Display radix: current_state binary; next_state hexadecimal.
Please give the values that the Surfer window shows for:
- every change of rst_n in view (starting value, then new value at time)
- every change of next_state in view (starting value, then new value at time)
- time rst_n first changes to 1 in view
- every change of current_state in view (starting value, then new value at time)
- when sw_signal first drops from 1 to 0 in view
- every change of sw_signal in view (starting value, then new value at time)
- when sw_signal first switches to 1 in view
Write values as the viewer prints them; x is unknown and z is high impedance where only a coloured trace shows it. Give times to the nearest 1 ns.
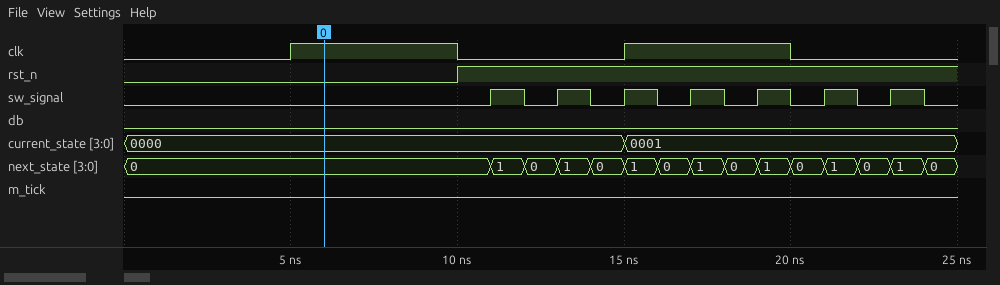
0, 1 at 10 ns
0, 1 at 11 ns, 0 at 12 ns, 1 at 13 ns, 0 at 14 ns, 1 at 15 ns, 0 at 16 ns, 1 at 17 ns, 0 at 18 ns, 1 at 19 ns, 0 at 20 ns, 1 at 21 ns, 0 at 22 ns, 1 at 23 ns, 0 at 24 ns
10 ns
0000, 0001 at 15 ns
12 ns
0, 1 at 11 ns, 0 at 12 ns, 1 at 13 ns, 0 at 14 ns, 1 at 15 ns, 0 at 16 ns, 1 at 17 ns, 0 at 18 ns, 1 at 19 ns, 0 at 20 ns, 1 at 21 ns, 0 at 22 ns, 1 at 23 ns, 0 at 24 ns
11 ns
